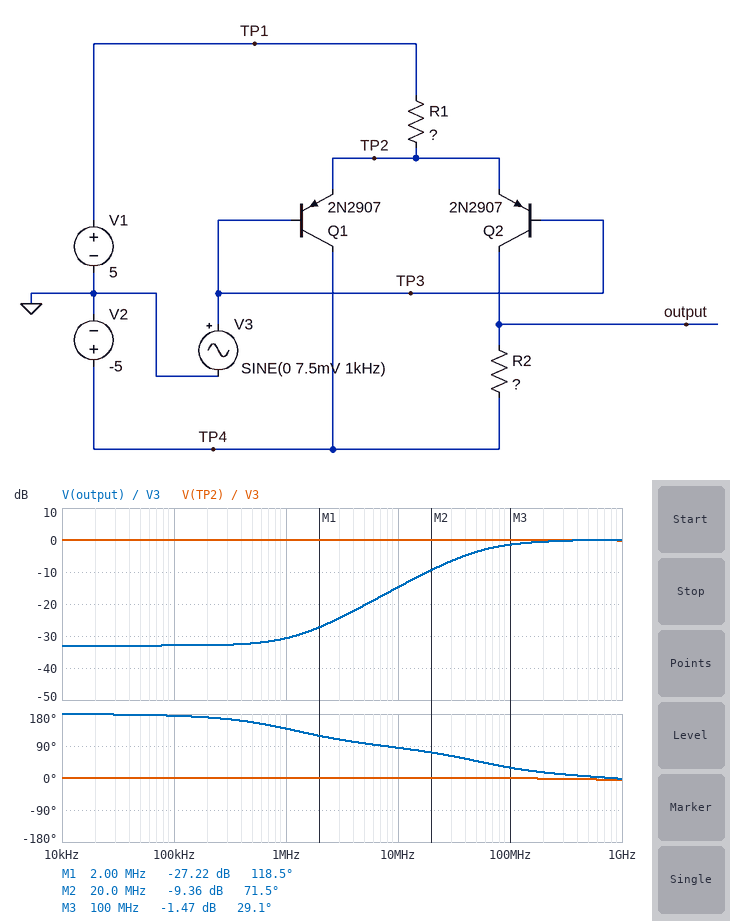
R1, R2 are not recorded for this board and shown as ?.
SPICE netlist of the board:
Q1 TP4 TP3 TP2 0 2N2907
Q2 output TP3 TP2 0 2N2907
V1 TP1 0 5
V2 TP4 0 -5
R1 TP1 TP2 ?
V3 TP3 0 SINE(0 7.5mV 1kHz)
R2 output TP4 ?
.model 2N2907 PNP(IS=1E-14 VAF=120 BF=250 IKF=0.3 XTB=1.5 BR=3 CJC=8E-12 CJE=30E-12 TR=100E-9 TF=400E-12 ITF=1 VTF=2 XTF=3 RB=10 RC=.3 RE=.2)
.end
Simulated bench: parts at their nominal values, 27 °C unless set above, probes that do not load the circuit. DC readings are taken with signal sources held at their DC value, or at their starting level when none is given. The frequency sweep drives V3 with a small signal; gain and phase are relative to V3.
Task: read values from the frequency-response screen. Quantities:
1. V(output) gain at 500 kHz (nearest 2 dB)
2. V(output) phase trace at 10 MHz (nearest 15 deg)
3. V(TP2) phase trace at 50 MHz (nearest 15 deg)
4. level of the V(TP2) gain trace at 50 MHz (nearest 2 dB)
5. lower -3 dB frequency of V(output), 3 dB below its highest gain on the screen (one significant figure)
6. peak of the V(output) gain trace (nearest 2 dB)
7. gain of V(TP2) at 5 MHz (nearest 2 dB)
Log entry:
-32 dB
90 deg
0 deg
0 dB
60 MHz
0 dB
0 dB
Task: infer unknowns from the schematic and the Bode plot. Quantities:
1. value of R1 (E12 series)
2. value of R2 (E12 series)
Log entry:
15 kΩ
680 Ω
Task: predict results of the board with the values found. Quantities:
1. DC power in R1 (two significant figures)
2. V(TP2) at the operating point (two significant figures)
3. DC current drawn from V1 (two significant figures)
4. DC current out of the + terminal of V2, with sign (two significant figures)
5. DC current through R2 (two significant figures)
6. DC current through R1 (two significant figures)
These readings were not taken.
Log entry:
1.3 mW
600 mV
290 µA
-290 µA
150 µA
290 µA
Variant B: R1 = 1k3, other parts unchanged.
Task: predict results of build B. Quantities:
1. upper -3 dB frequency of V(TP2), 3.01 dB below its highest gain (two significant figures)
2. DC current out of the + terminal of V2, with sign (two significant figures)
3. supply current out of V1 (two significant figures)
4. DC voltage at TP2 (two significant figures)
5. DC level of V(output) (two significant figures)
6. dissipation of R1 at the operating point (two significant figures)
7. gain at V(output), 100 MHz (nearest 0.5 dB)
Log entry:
7.4 GHz
-3.3 mA
3.3 mA
670 mV
-3.9 V
14 mW
-2.5 dB
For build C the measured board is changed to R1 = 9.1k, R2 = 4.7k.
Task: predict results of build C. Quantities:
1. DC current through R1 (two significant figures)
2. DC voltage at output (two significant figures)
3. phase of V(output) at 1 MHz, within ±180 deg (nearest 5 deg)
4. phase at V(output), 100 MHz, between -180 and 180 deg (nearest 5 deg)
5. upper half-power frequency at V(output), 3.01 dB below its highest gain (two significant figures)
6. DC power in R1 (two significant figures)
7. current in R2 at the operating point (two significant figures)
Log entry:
480 µA
-3.9 V
145 deg
5 deg
7.8 GHz
2.1 mW
240 µA
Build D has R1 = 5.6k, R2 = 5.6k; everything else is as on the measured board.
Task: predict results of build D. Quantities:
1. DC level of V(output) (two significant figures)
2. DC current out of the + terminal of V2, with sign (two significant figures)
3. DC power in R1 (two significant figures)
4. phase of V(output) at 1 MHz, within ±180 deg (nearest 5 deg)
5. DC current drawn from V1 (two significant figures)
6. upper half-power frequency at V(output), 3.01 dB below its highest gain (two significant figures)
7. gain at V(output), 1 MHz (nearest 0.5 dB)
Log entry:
-2.8 V
-780 µA
3.4 mW
150 deg
780 µA
7.8 GHz
-6.0 dB
